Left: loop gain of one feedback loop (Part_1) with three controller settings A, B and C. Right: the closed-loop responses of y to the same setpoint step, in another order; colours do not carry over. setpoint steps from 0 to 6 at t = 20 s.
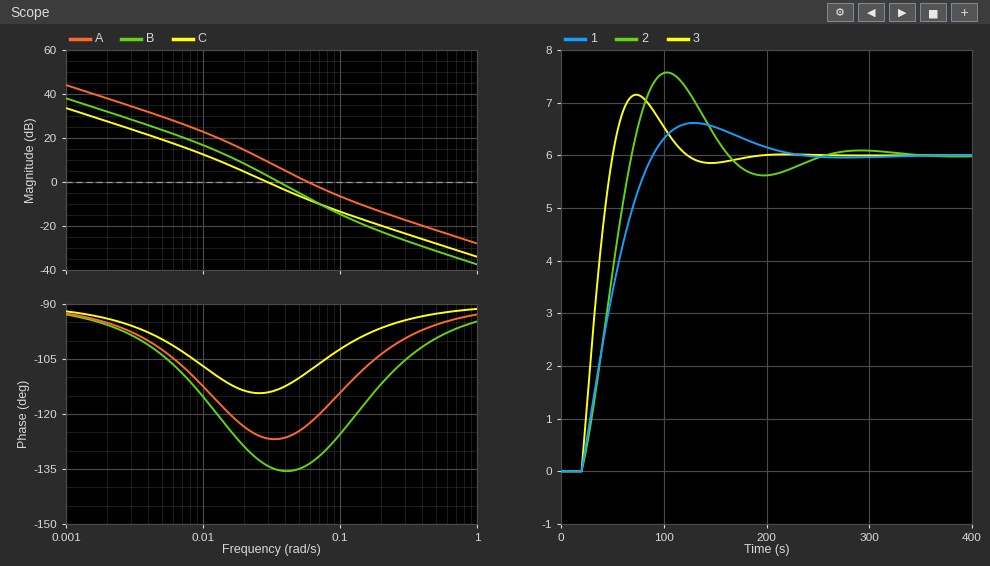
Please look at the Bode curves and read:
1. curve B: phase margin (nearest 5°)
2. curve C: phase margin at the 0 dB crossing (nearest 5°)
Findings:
45°
65°
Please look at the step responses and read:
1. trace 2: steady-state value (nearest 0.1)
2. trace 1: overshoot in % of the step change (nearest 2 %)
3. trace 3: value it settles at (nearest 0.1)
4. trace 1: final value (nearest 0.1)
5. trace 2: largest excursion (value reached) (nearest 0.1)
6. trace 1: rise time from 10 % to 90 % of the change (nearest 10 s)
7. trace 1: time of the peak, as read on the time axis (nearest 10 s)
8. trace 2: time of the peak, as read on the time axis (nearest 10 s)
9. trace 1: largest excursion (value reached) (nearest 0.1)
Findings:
6.0
10 %
6.0
6.0
7.6
50 s
130 s
100 s
6.6
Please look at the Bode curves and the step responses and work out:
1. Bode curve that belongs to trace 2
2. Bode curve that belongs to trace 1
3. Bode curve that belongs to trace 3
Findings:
B
C
A
